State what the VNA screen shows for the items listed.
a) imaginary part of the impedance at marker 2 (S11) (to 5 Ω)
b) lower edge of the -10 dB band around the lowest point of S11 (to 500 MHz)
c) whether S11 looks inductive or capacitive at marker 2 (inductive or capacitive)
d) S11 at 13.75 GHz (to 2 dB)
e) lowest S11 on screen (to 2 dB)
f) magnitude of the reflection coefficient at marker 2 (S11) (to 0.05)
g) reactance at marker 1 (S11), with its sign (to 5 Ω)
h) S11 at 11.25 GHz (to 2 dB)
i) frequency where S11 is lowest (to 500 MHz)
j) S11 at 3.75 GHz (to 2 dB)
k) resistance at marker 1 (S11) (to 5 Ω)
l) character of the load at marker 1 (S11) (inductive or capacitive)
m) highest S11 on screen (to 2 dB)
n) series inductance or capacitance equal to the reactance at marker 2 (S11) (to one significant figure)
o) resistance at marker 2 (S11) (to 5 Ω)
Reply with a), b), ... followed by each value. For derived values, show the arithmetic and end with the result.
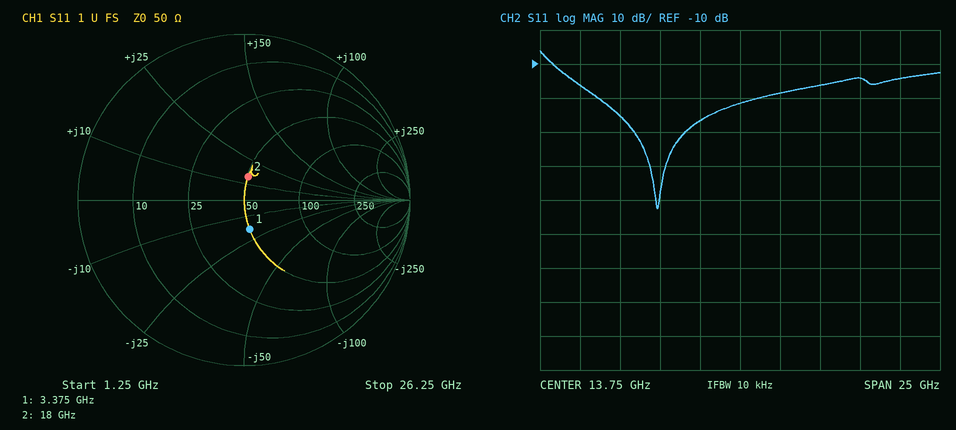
a) +15 Ω
b) 2.0 GHz
c) inductive
d) -22 dB
e) -52 dB
f) 0.15
g) -20 Ω
h) -26 dB
i) 8.5 GHz
j) -16 dB
k) 50 Ω
l) capacitive
m) -6 dB
n) L = 15 Ω/(2π × 18 GHz) ≈ 133 pH, so 100 pH to one significant figure
o) 50 Ω
